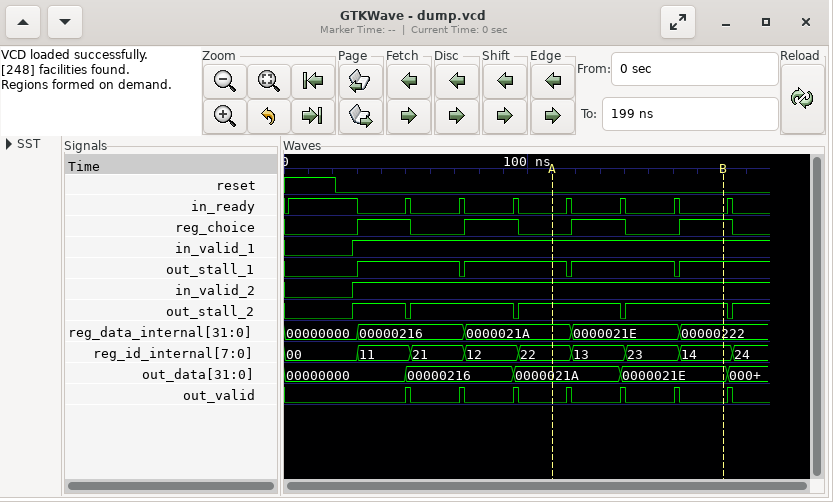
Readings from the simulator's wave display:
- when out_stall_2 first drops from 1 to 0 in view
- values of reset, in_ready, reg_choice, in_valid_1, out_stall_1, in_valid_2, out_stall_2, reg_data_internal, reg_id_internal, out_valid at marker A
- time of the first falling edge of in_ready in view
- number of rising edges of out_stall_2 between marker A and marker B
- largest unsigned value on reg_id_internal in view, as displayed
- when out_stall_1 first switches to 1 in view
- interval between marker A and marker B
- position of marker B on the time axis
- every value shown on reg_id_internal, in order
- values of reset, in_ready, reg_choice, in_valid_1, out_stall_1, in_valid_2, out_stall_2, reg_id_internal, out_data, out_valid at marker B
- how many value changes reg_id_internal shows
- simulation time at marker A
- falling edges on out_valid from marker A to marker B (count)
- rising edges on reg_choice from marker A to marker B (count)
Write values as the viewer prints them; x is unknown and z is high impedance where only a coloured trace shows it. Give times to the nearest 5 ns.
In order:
50 ns
reset=0, in_ready=0, reg_choice=0, in_valid_1=1, out_stall_1=1, in_valid_2=1, out_stall_2=1, reg_data_internal=0000021A, reg_id_internal=22, out_valid=0
30 ns
1
24
30 ns
70 ns
180 ns
00, 11, 21, 12, 22, 13, 23, 14, 24
reset=0, in_ready=0, reg_choice=1, in_valid_1=1, out_stall_1=1, in_valid_2=1, out_stall_2=1, reg_id_internal=14, out_data=0000021E, out_valid=0
8
110 ns
3
2
